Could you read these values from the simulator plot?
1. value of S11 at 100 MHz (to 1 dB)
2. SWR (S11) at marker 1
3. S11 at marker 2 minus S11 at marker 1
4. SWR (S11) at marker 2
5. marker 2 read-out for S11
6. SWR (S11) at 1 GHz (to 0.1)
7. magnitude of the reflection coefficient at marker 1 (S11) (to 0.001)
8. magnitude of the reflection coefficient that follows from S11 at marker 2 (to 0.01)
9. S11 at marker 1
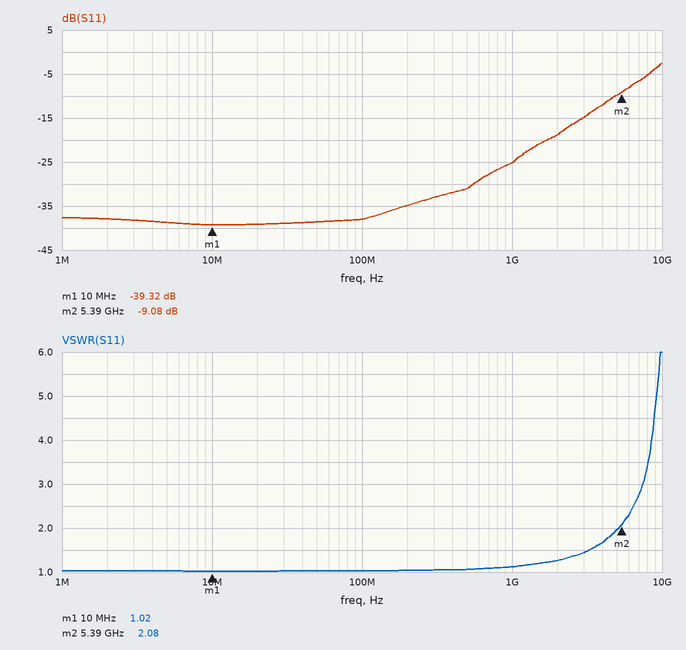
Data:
-38 dB
1.02
30.24 dB
2.08
-9.08 dB
1.1
0.011
0.35
-39.32 dB
